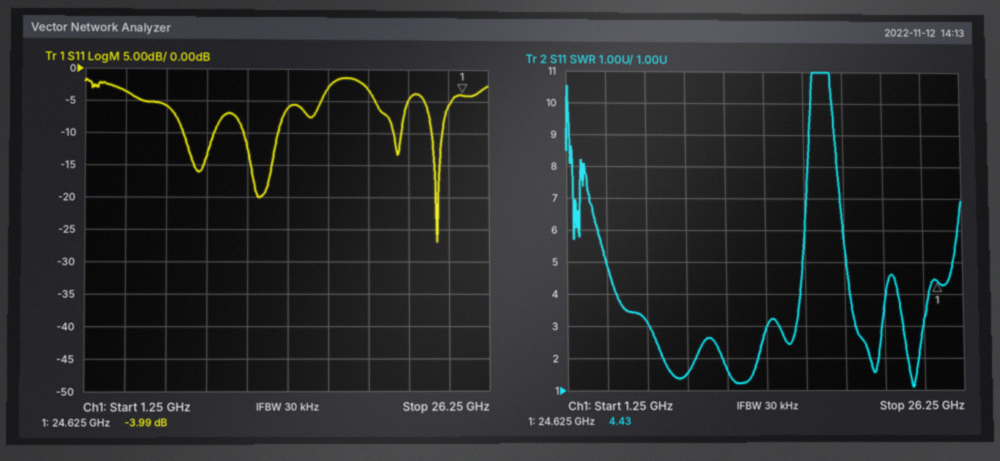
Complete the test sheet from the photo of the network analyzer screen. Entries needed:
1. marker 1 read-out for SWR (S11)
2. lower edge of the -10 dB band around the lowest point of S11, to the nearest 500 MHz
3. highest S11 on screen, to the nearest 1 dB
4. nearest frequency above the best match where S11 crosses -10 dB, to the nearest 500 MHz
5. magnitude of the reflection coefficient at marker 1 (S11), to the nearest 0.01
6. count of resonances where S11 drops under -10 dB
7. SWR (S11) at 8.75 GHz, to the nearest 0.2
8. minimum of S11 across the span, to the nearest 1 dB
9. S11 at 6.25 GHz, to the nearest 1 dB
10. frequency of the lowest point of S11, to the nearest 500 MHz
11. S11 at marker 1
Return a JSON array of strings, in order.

["4.43", "22.5 GHz", "-1 dB", "23.5 GHz", "0.63", "4", "1.6", "-27 dB", "-6 dB", "23.0 GHz", "-3.99 dB"]
